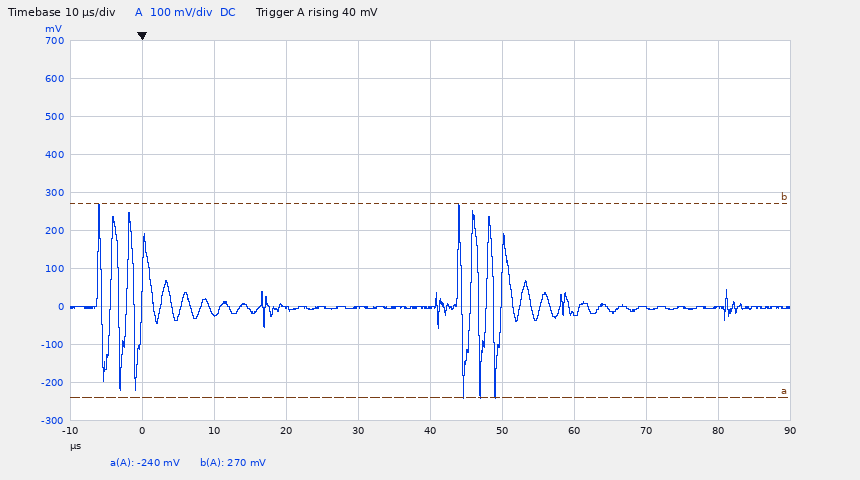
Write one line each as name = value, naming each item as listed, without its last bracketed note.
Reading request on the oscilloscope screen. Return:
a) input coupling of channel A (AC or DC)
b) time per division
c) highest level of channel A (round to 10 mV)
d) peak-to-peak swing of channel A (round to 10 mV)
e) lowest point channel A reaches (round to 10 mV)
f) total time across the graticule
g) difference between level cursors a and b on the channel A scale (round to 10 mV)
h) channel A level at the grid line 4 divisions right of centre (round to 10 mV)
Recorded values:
input coupling of channel A = DC
time per division = 10 µs
highest level of channel A = 270 mV
peak-to-peak swing of channel A = 510 mV
lowest point channel A reaches = -240 mV
total time across the graticule = 100 µs
difference between level cursors a and b on the channel A scale = 510 mV
channel A level at the grid line 4 divisions right of centre = 0 mV
